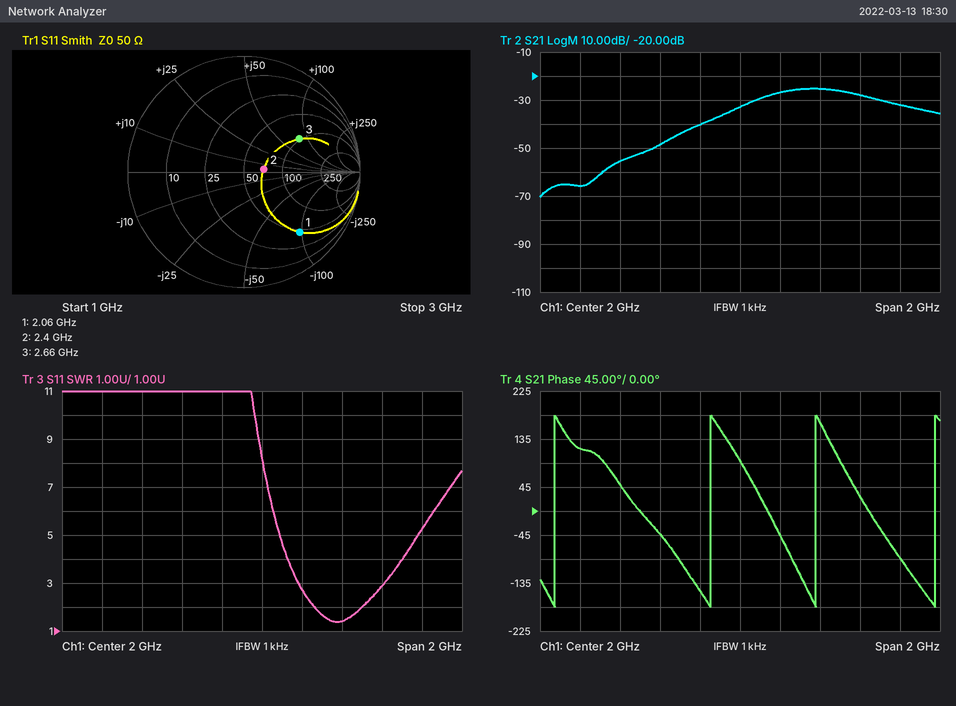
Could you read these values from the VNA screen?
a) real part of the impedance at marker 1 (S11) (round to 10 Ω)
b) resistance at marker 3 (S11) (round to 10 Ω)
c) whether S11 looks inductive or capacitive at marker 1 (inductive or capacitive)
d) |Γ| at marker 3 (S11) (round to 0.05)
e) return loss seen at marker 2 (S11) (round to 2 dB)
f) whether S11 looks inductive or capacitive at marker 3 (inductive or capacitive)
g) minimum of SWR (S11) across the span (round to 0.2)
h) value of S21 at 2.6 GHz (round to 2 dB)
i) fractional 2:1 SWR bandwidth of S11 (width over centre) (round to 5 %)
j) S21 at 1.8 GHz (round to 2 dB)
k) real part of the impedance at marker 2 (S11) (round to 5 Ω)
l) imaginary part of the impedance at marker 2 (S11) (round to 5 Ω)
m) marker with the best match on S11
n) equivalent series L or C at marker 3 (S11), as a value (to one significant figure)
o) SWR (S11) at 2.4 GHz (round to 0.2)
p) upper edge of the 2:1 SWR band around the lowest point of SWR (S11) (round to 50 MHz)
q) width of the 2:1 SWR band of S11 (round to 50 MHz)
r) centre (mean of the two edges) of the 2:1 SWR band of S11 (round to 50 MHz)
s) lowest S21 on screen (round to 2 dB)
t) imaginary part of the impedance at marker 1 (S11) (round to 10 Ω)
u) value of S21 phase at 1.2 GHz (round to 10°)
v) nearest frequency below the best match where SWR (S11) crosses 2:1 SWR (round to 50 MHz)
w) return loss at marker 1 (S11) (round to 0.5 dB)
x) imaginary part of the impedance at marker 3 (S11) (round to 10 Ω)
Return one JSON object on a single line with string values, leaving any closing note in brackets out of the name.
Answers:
{"real part of the impedance at marker 1 (S11)": "50 Ω", "resistance at marker 3 (S11)": "100 Ω", "whether S11 looks inductive or capacitive at marker 1": "capacitive", "|Γ| at marker 3 (S11)": "0.55", "return loss seen at marker 2 (S11)": "16 dB", "whether S11 looks inductive or capacitive at marker 3": "inductive", "minimum of SWR (S11) across the span": "1.4", "value of S21 at 2.6 GHz": "-28 dB", "fractional 2:1 SWR bandwidth of S11 (width over centre)": "10 %", "S21 at 1.8 GHz": "-40 dB", "real part of the impedance at marker 2 (S11)": "70 Ω", "imaginary part of the impedance at marker 2 (S11)": "+5 Ω", "marker with the best match on S11": "marker 2", "equivalent series L or C at marker 3 (S11), as a value": "5 nH", "SWR (S11) at 2.4 GHz": "1.4", "upper edge of the 2:1 SWR band around the lowest point of SWR (S11)": "2.50 GHz", "width of the 2:1 SWR band of S11": "250 MHz", "centre (mean of the two edges) of the 2:1 SWR band of S11": "2.40 GHz", "lowest S21 on screen": "-70 dB", "imaginary part of the impedance at marker 1 (S11)": "-100 Ω", "value of S21 phase at 1.2 GHz": "120°", "nearest frequency below the best match where SWR (S11) crosses 2:1 SWR": "2.25 GHz", "return loss at marker 1 (S11)": "3.0 dB", "imaginary part of the impedance at marker 3 (S11)": "+80 Ω"}
